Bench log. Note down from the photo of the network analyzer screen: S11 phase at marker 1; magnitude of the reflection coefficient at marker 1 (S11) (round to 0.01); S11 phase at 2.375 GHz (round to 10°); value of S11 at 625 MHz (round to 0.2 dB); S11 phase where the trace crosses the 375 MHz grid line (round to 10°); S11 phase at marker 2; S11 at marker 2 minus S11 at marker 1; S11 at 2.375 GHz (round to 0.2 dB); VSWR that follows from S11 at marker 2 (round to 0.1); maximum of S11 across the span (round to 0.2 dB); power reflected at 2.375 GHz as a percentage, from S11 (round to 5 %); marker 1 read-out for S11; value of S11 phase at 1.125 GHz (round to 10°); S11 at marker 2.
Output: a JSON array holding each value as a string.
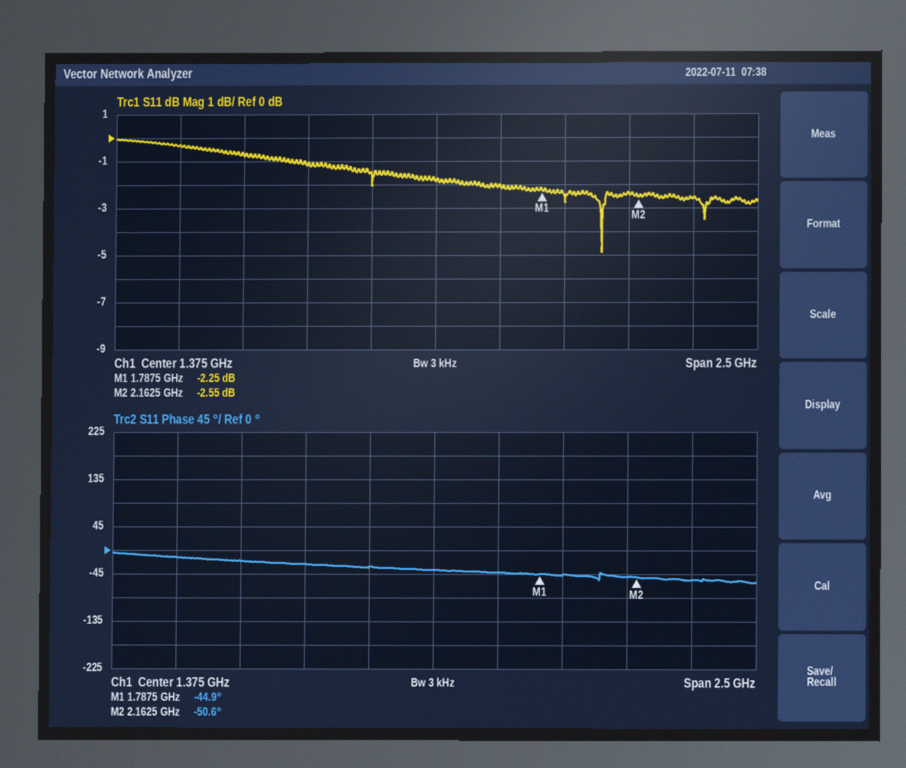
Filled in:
["-44.9°", "0.77", "-60°", "-0.8 dB", "-10°", "-50.6°", "-0.30 dB", "-2.6 dB", "6.9", "0.0 dB", "55 %", "-2.25 dB", "-30°", "-2.55 dB"]
